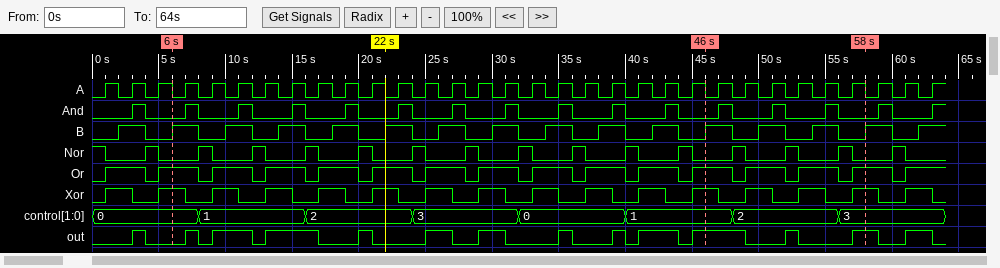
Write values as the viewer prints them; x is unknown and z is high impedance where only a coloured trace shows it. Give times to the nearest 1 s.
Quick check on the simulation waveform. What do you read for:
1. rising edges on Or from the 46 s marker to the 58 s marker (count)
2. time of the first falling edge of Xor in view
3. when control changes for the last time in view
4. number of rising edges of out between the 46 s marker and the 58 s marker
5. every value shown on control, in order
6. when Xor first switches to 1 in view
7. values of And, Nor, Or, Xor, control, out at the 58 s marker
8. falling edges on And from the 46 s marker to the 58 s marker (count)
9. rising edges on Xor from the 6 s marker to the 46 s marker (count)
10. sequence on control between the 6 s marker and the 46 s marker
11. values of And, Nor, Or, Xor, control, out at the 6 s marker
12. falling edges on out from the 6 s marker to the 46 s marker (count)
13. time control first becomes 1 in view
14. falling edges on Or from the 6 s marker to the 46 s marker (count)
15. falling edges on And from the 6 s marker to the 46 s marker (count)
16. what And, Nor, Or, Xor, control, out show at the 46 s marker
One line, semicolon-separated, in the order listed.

3; 3 s; 56 s; 2; 0, 1, 2, 3, 0, 1, 2, 3; 1 s; And=0, Nor=0, Or=1, Xor=1, control=3, out=1; 3; 10; 0, 1, 2, 3, 0, 1; And=0, Nor=0, Or=1, Xor=1, control=0, out=0; 9; 8 s; 10; 10; And=0, Nor=0, Or=1, Xor=1, control=1, out=1
